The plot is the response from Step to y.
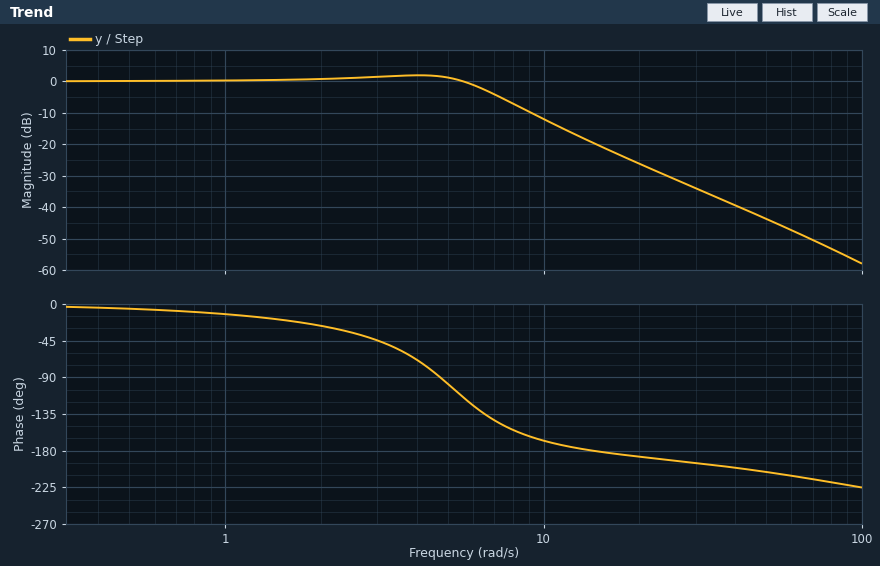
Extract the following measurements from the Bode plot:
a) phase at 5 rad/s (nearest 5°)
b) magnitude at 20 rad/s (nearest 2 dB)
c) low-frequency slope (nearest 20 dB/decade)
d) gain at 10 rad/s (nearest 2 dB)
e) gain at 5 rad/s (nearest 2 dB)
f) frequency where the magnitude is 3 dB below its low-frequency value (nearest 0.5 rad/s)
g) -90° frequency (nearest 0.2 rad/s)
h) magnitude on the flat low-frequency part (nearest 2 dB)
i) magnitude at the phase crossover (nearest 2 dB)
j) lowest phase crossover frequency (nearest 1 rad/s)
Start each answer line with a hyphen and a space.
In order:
- -100°
- -26 dB
- 0 dB/decade
- -12 dB
- 2 dB
- 6.5 rad/s
- 4.8 rad/s
- 0 dB
- -20 dB
- 14 rad/s
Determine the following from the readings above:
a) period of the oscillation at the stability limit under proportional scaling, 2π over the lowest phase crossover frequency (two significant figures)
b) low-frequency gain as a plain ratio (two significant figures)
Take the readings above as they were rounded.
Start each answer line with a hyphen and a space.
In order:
- 0.45 s
- 1.0
